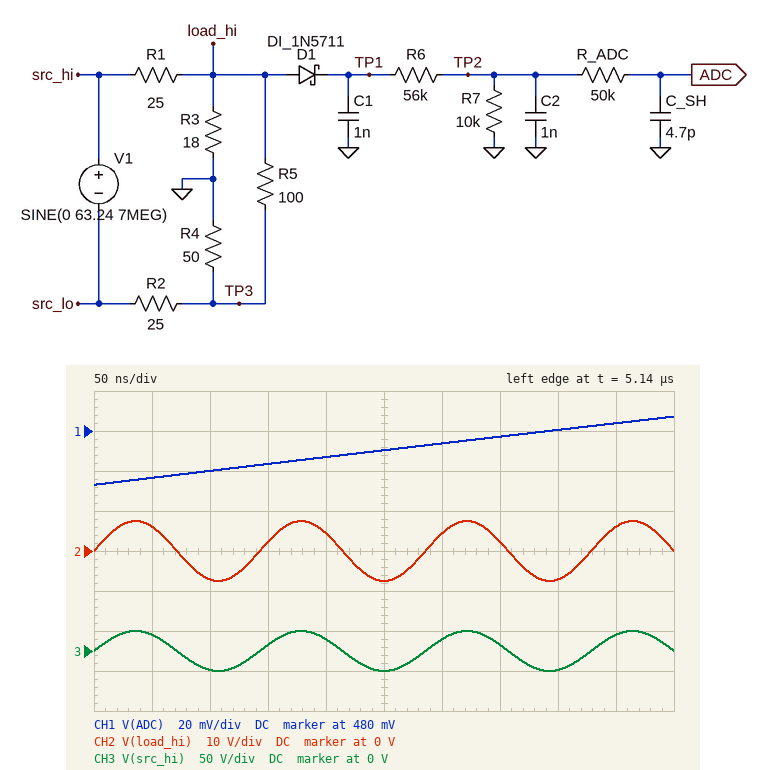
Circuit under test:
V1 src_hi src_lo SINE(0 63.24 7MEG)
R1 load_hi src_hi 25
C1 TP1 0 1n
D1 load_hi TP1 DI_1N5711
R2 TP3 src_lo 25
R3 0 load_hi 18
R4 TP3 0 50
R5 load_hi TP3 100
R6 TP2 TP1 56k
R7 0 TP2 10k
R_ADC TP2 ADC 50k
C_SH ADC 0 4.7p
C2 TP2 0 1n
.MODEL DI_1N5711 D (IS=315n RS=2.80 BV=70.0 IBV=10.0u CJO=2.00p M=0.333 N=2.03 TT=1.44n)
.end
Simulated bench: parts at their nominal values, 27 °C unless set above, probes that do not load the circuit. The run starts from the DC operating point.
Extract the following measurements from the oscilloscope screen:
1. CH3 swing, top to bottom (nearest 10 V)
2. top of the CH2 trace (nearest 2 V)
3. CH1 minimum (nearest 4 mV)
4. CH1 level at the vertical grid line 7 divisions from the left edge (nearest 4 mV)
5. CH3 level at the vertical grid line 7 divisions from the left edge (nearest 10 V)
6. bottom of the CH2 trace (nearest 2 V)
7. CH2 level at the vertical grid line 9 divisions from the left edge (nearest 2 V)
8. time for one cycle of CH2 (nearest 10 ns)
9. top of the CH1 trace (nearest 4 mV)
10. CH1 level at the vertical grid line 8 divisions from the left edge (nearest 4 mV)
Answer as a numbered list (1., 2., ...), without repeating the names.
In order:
1. 50 V
2. 8 V
3. 452 mV
4. 476 mV
5. 10 V
6. -8 V
7. 6 V
8. 140 ns
9. 488 mV
10. 480 mV
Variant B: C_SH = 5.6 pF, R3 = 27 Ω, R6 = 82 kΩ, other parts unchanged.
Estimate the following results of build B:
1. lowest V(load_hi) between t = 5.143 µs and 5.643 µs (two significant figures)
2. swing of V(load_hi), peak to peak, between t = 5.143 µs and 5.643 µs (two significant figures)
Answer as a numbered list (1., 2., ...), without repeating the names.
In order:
1. -10 V
2. 21 V
